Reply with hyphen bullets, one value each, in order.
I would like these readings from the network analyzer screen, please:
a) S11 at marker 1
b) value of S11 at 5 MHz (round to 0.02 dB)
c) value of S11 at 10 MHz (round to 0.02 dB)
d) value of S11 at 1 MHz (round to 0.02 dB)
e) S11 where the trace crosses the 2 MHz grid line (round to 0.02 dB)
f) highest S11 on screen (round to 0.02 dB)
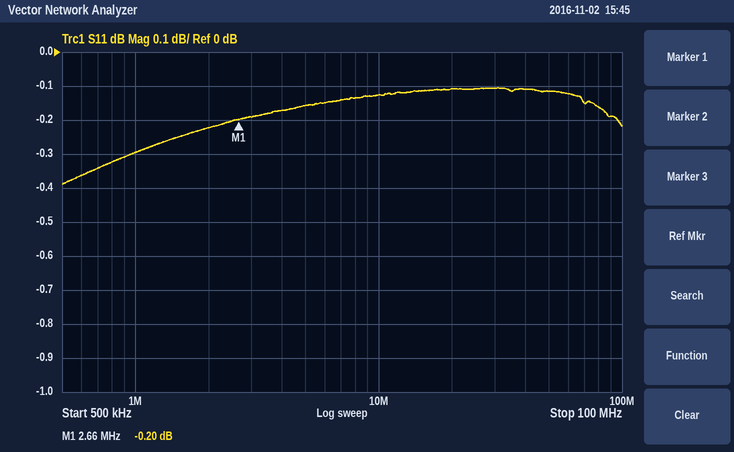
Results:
- -0.20 dB
- -0.16 dB
- -0.12 dB
- -0.30 dB
- -0.22 dB
- -0.10 dB
